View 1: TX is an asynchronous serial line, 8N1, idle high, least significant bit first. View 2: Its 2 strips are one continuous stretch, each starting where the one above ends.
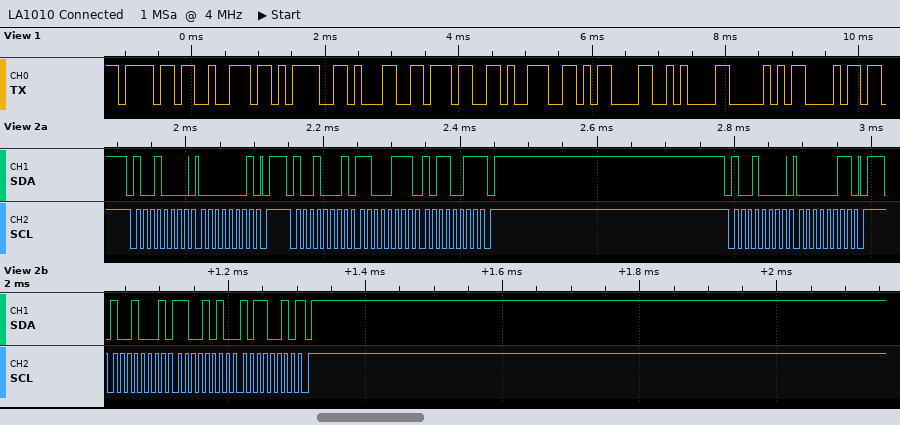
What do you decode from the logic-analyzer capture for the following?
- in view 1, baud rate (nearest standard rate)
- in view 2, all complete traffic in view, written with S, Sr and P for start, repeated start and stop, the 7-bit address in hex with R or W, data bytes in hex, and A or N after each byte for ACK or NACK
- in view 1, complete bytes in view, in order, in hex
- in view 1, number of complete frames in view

9600 baud
S 48W A 01 A P S 48R A C7 A B3 N P S 48W A 03 A P S 48R A CA A B2 N P
6F 72 3D 31 37 39 0D 0A 50 68
10
